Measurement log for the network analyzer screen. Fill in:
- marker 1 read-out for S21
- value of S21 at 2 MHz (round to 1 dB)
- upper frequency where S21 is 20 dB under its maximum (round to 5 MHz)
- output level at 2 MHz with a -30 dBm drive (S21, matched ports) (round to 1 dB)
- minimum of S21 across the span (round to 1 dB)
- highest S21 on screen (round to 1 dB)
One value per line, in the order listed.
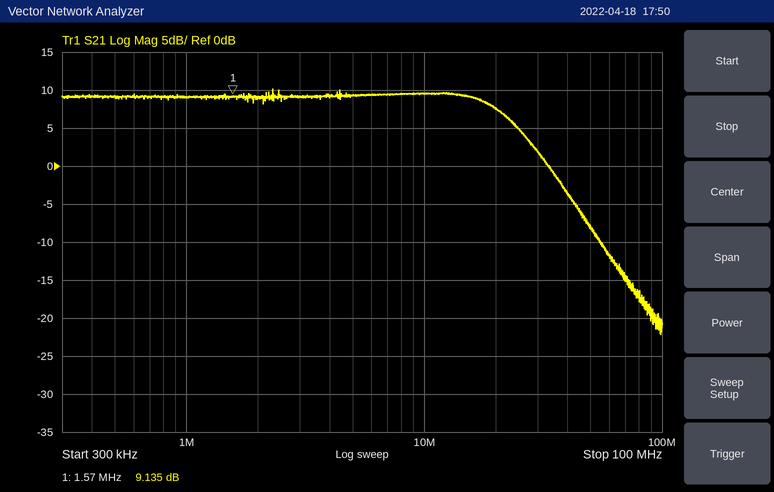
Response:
9.135 dB
9 dB
55 MHz
-21 dBm
-22 dB
10 dB
